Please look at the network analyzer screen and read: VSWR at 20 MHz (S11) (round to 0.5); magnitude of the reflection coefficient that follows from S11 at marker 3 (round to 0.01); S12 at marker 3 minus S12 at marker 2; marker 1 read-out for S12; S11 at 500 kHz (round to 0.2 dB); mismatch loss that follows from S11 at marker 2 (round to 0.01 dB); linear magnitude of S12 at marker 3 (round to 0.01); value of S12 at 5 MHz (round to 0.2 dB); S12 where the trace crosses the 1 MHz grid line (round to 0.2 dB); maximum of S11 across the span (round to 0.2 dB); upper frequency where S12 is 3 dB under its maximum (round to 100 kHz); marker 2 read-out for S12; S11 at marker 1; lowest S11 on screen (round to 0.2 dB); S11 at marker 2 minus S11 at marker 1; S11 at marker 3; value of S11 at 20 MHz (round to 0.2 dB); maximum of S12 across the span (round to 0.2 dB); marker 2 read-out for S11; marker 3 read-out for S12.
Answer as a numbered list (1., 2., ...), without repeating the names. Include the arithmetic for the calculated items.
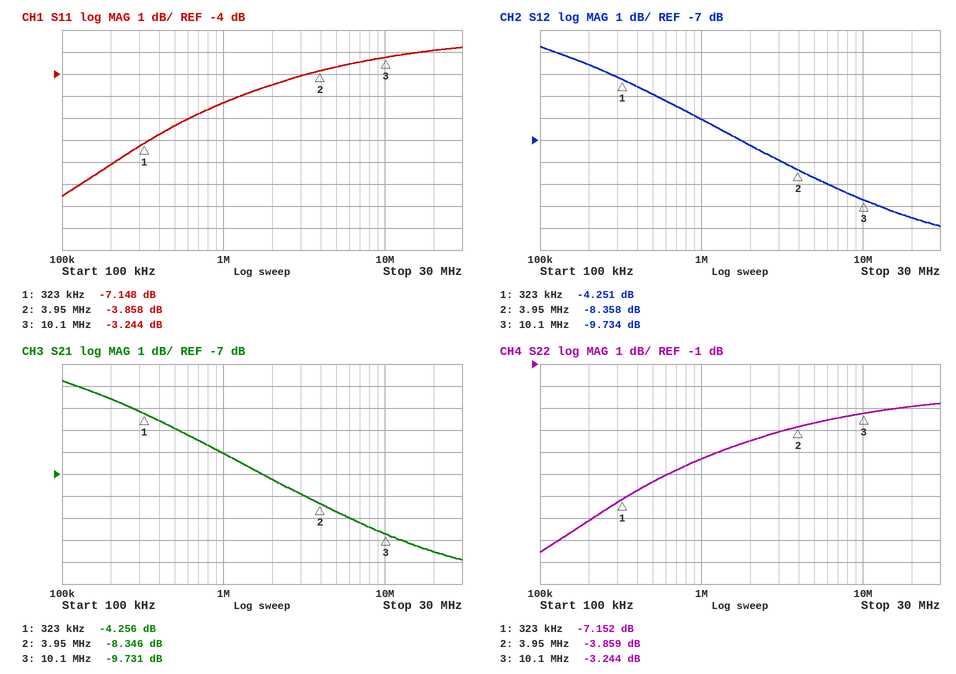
1. |Γ| = 10^(-3/20) = 0.7079; VSWR = (1 + 0.7079)/(1 − 0.7079) ≈ 5.85, so 6.0 to the nearest 0.5
2. 10^(-3.244/20) ≈ 0.69
3. -9.734 − (-8.358) = -1.376 dB
4. -4.251 dB
5. -6.4 dB
6. −10 log10(1 − 10^(-3.858/10)) ≈ 2.30 dB
7. 10^(-9.734/20) ≈ 0.33
8. -8.8 dB
9. -6.0 dB
10. -2.8 dB
11. 800 kHz
12. -8.358 dB
13. -7.148 dB
14. -9.6 dB
15. -3.858 − (-7.148) = 3.290 dB
16. -3.244 dB
17. -3.0 dB
18. -2.8 dB
19. -3.858 dB
20. -9.734 dB
